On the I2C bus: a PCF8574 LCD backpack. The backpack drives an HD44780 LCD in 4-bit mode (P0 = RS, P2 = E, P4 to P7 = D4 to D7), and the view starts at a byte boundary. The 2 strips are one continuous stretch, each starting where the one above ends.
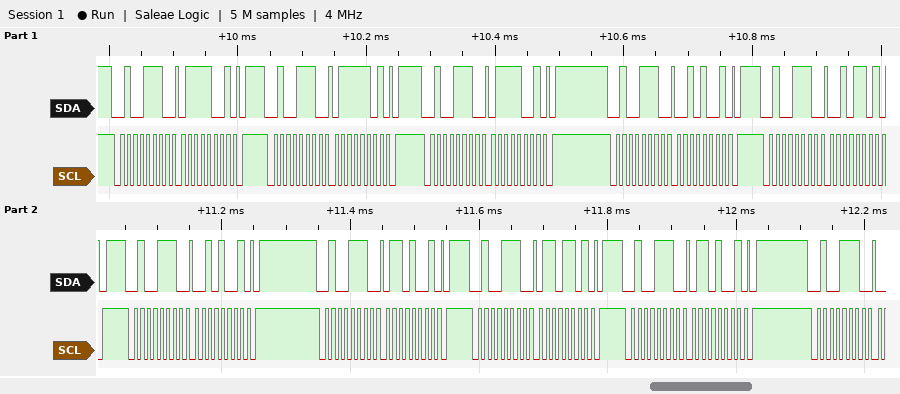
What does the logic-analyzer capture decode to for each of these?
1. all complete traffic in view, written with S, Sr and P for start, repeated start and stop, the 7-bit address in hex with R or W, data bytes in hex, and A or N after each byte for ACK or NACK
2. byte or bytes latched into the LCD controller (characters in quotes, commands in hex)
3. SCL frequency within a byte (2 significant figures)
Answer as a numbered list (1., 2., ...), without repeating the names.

1. S 27W A 79 A P S 27W A 7D A P S 27W A 79 A P S 27W A 29 A P S 27W A 2D A P S 27W A 29 A P S 27W A 69 A P S 27W A 6D A P S 27W A 69 A P S 27W A
2. 'r'
3. 100 kHz
